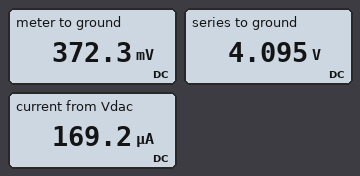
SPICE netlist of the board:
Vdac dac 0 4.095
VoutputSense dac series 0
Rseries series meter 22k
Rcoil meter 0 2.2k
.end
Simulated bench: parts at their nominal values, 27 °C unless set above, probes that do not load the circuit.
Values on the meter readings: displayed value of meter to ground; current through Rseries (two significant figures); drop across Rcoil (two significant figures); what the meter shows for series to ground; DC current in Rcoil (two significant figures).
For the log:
372.3 mV
170 µA
370 mV
4.095 V
170 µA
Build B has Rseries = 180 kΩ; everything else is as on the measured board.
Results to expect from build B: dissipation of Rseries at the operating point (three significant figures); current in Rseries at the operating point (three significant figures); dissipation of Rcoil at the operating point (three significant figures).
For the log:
90.9 µW
22.5 µA
1.11 µW
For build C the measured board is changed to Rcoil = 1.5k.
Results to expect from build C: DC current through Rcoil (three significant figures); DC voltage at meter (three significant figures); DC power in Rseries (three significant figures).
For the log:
174 µA
261 mV
668 µW
